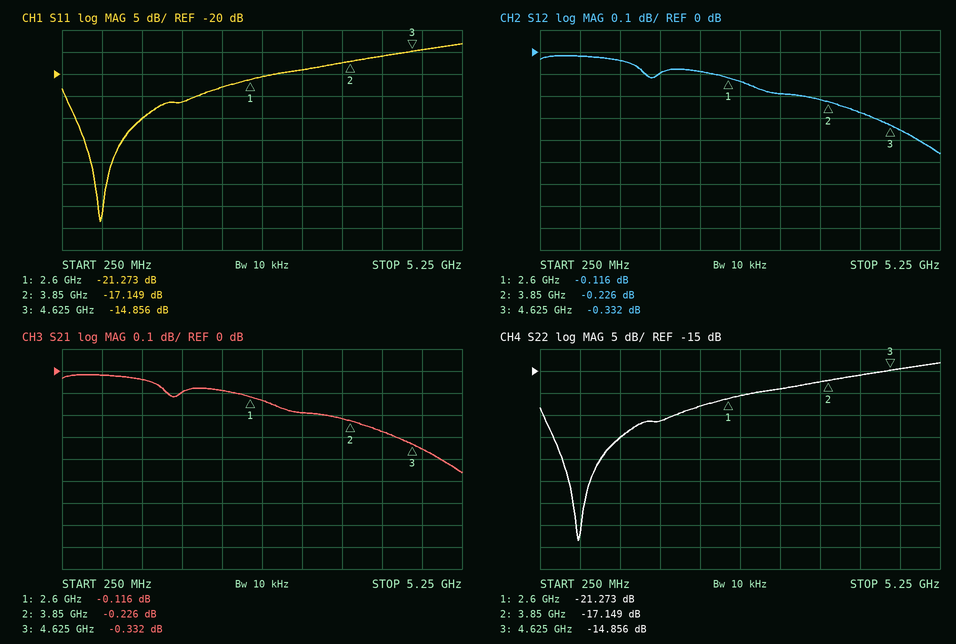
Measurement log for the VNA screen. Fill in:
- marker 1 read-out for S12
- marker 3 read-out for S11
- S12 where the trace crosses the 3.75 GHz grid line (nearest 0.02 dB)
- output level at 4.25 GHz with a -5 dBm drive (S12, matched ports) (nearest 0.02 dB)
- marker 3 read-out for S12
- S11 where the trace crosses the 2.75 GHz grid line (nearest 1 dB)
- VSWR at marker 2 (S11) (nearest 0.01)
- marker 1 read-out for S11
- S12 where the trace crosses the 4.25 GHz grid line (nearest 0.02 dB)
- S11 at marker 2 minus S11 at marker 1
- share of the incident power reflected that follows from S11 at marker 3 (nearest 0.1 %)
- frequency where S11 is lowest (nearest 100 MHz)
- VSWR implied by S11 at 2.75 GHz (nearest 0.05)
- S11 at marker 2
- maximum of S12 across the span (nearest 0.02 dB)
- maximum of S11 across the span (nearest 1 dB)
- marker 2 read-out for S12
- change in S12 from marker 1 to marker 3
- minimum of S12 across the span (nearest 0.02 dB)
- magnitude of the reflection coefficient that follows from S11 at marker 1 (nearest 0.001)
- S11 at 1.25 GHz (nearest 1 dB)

-0.116 dB
-14.856 dB
-0.22 dB
-5.28 dBm
-0.332 dB
-21 dB
1.32
-21.273 dB
-0.28 dB
4.124 dB
3.3 %
700 MHz
1.20
-17.149 dB
-0.02 dB
-13 dB
-0.226 dB
-0.216 dB
-0.46 dB
0.086
-30 dB
